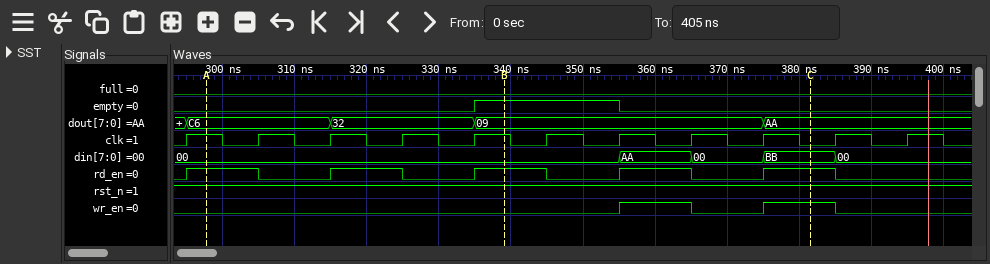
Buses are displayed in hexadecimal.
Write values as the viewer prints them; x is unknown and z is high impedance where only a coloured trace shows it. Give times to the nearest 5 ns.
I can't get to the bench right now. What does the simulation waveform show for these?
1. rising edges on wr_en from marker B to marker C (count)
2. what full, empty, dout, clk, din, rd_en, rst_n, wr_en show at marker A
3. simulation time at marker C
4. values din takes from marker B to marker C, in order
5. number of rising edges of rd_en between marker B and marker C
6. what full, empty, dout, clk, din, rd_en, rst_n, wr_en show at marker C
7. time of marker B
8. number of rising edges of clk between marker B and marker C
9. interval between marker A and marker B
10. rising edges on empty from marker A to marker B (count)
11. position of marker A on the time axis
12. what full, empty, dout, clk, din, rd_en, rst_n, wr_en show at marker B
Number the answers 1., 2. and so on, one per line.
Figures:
1. 2
2. full=0, empty=0, dout=C6, clk=1, din=00, rd_en=1, rst_n=1, wr_en=0
3. 380 ns
4. 00, AA, 00, BB
5. 2
6. full=0, empty=0, dout=AA, clk=0, din=BB, rd_en=1, rst_n=1, wr_en=1
7. 340 ns
8. 4
9. 40 ns
10. 1
11. 300 ns
12. full=0, empty=1, dout=09, clk=1, din=00, rd_en=1, rst_n=1, wr_en=0
